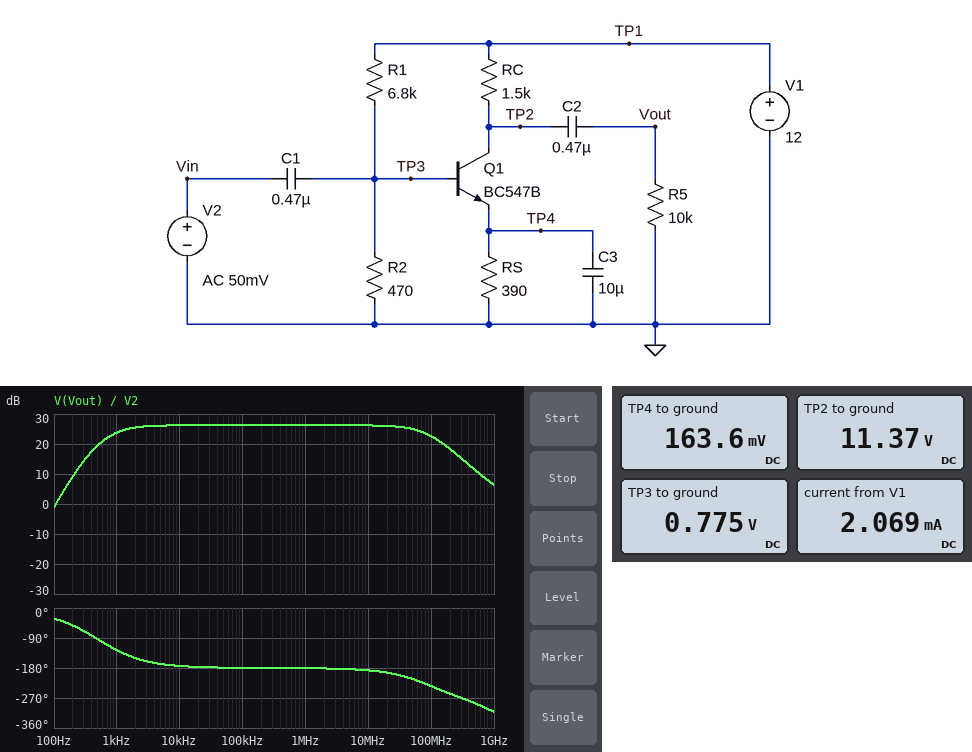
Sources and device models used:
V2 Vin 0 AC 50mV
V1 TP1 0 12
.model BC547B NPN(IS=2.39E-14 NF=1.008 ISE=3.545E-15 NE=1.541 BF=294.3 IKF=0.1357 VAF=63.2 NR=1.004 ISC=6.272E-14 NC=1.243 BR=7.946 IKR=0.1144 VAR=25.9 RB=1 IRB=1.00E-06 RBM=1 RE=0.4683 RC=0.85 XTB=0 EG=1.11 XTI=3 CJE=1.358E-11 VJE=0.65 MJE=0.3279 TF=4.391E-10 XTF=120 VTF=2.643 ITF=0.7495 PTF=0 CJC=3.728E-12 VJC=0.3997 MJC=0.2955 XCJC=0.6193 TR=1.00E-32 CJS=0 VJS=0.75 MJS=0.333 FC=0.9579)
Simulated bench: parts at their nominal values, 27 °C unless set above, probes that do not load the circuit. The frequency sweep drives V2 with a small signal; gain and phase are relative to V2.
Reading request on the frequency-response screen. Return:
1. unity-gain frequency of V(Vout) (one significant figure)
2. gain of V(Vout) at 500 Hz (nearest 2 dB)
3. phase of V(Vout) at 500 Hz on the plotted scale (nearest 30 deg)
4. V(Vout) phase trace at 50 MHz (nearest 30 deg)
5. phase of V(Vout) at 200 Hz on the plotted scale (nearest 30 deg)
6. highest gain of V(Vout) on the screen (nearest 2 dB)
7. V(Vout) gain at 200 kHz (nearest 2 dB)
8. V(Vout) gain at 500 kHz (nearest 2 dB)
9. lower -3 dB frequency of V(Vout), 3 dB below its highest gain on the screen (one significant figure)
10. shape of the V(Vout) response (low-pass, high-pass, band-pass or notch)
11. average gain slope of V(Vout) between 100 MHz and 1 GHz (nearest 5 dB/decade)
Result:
100 Hz
20 dB
-90 deg
-210 deg
-60 deg
26 dB
26 dB
26 dB
900 Hz
band-pass
-15 dB/decade
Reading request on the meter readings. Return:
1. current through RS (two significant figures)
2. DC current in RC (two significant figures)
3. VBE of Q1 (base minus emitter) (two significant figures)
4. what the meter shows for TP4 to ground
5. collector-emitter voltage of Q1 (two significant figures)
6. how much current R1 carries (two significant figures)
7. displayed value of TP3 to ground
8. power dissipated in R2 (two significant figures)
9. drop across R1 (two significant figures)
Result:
420 µA
420 µA
610 mV
163.6 mV
11 V
1.7 mA
0.775 V
1.3 mW
11 V
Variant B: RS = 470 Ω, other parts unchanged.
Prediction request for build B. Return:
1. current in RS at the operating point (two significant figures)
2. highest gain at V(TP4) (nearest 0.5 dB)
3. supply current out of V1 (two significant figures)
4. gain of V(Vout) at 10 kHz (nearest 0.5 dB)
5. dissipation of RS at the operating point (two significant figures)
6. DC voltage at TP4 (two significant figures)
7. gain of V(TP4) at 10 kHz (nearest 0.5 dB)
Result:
360 µA
-13.5 dB
2.0 mA
25.0 dB
60 µW
170 mV
-33.5 dB
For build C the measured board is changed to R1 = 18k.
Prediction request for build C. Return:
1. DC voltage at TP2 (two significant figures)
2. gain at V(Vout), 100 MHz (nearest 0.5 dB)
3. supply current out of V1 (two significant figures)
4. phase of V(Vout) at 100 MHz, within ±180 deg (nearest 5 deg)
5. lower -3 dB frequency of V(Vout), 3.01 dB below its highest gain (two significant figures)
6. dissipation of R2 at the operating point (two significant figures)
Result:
12 V
-2.5 dB
650 µA
40 deg
88 MHz
200 µW
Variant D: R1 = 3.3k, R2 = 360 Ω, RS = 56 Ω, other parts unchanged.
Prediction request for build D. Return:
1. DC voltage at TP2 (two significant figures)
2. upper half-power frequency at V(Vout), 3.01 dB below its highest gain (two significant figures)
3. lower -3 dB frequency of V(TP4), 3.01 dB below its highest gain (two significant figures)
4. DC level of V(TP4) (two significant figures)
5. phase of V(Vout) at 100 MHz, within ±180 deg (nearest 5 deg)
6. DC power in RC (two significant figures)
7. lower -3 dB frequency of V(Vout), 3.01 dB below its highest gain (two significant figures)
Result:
520 mV
76 MHz
320 Hz
440 mV
110 deg
88 mW
15 kHz
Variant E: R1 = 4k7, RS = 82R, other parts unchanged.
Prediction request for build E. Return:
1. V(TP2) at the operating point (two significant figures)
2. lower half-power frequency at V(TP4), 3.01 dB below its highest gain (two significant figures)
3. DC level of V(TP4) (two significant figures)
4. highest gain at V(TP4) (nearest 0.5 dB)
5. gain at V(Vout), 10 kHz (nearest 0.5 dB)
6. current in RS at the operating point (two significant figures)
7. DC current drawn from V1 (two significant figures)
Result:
4.7 V
510 Hz
400 mV
-3.5 dB
45.5 dB
4.9 mA
7.2 mA
